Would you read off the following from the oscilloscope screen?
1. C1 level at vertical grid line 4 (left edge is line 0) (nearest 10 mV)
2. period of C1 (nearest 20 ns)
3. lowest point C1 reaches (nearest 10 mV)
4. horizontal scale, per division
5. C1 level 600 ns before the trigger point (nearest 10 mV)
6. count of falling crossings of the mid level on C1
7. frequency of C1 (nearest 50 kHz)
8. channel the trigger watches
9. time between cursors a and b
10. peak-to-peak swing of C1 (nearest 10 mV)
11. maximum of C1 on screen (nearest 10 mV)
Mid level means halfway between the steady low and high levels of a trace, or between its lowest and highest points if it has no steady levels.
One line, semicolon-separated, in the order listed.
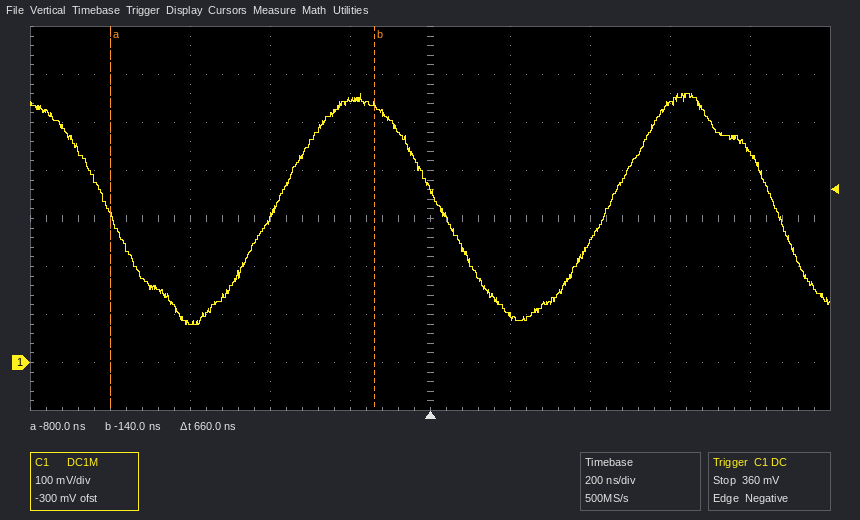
550 mV; 840 ns; 80 mV; 200 ns; 80 mV; 3; 1.20 MHz; C1; 660 ns; 480 mV; 560 mV
